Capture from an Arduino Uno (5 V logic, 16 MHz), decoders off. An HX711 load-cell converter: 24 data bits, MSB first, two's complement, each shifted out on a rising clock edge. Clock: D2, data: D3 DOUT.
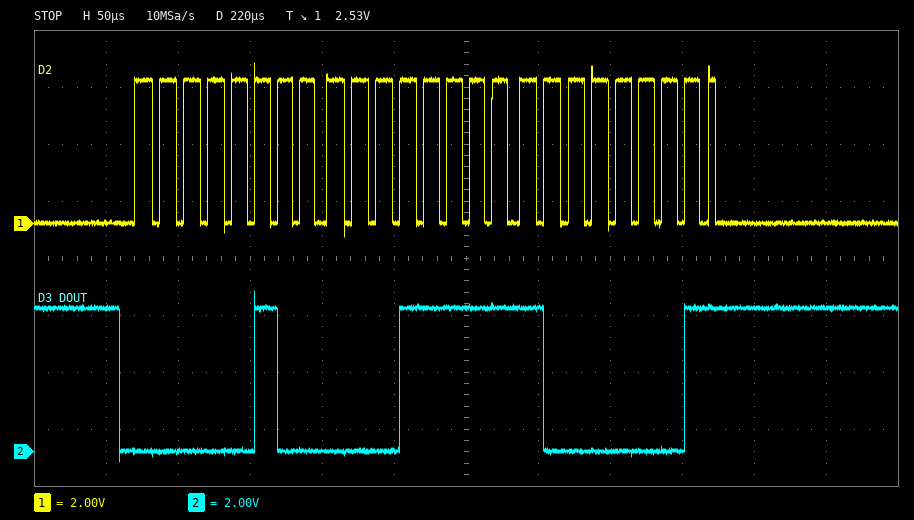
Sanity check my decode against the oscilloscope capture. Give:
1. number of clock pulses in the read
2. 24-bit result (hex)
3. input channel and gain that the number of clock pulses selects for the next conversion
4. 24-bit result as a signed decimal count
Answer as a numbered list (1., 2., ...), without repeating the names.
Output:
1. 25
2. 0x041F81
3. channel A, gain 128
4. 270209
